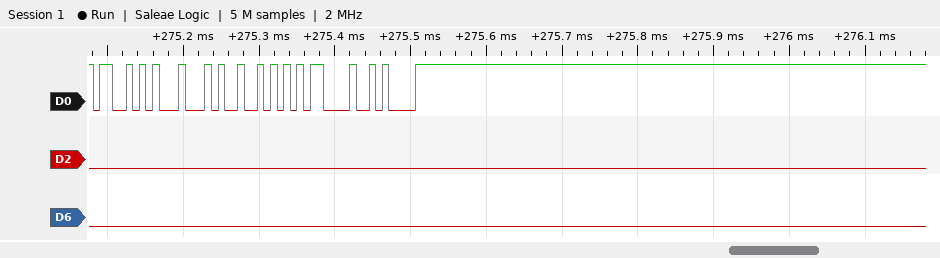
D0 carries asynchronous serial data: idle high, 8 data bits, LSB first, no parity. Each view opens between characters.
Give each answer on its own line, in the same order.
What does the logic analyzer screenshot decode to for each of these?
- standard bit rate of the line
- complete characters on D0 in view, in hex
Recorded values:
115200 baud
53, 44, 52, 0D, 0A
